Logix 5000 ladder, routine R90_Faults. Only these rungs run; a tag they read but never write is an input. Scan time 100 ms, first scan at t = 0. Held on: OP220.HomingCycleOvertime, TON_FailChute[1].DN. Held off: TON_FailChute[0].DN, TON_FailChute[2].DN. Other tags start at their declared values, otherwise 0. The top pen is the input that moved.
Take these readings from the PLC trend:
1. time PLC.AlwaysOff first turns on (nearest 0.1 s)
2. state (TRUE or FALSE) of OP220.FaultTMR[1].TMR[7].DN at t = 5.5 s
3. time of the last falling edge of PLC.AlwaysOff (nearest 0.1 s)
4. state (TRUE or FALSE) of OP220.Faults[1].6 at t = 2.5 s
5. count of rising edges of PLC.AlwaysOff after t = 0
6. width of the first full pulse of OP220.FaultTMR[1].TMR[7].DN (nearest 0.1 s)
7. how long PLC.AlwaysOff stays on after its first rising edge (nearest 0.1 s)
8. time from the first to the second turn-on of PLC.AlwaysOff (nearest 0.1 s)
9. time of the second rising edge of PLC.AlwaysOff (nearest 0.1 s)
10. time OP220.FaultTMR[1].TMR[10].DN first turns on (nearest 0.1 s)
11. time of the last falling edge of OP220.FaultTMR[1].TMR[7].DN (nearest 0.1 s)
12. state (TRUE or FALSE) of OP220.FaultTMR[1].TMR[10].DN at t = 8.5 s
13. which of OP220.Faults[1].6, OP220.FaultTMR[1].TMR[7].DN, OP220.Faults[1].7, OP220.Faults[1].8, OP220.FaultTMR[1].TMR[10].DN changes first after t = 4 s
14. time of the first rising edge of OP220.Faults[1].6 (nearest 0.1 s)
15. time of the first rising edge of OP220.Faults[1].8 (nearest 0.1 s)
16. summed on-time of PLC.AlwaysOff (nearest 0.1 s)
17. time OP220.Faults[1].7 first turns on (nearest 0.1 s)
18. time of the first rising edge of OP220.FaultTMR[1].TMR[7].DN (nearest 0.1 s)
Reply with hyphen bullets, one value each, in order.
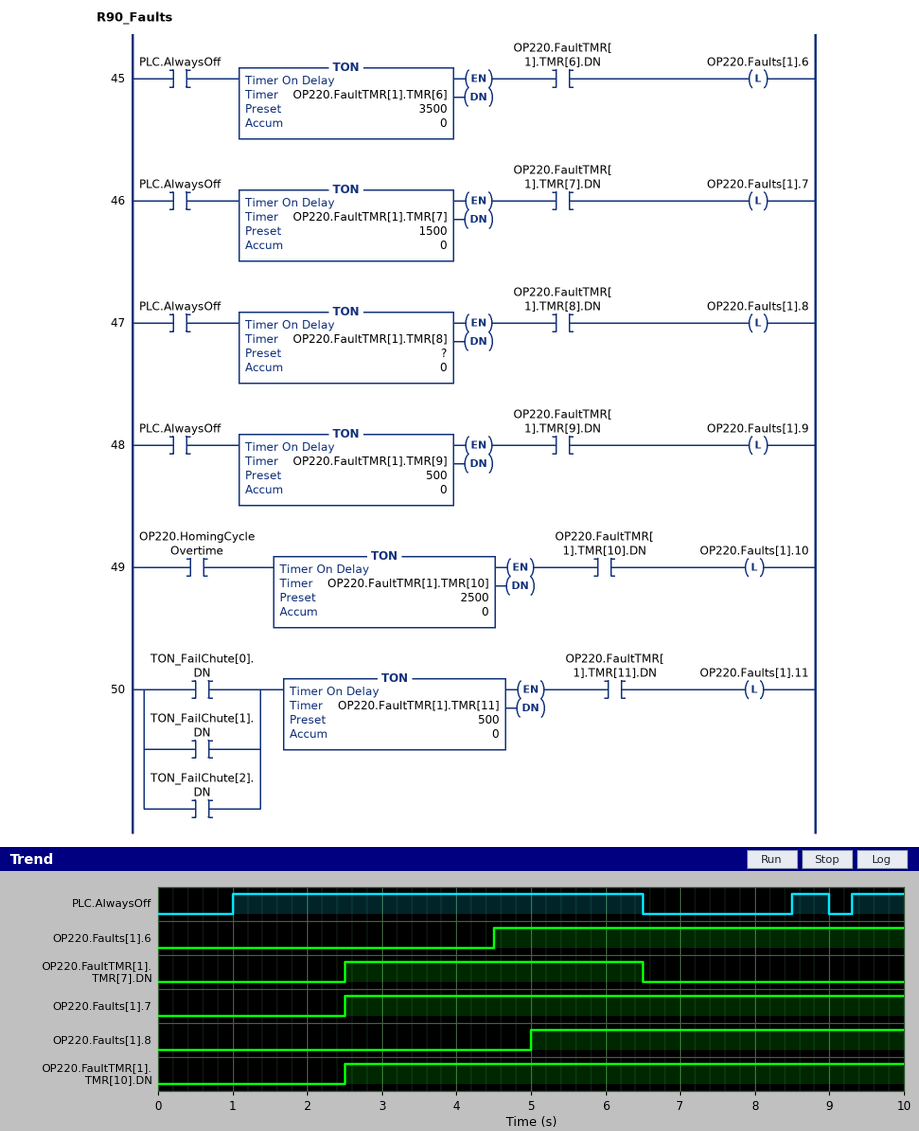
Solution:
- 1.0 s
- TRUE
- 9.0 s
- FALSE
- 3
- 4.0 s
- 5.5 s
- 7.5 s
- 8.5 s
- 2.5 s
- 6.5 s
- TRUE
- OP220.Faults[1].6
- 4.5 s
- 5.0 s
- 6.7 s
- 2.5 s
- 2.5 s
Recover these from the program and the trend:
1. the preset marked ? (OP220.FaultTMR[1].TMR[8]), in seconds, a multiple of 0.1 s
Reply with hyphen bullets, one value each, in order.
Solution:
- 4.0 s
